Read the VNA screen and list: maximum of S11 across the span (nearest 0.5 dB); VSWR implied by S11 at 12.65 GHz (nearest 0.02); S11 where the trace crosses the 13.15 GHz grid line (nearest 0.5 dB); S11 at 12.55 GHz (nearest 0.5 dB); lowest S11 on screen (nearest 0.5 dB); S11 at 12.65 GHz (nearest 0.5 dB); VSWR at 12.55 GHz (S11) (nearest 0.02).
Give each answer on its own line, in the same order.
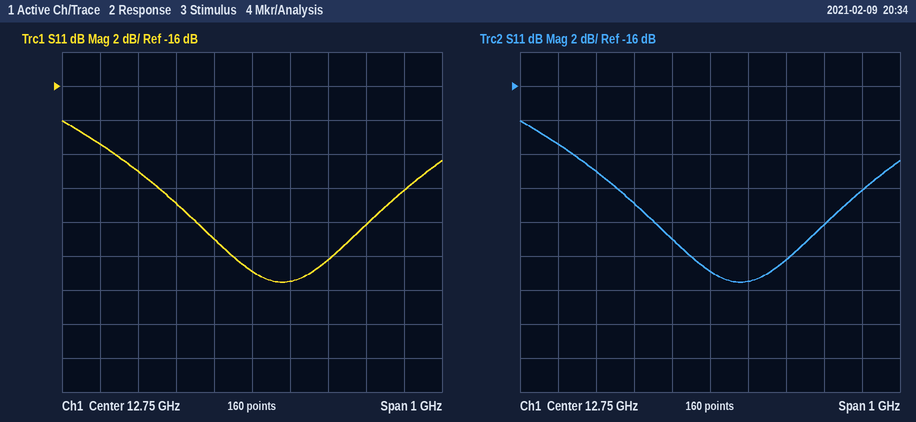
-18.0 dB
1.12
-22.0 dB
-23.0 dB
-27.5 dB
-25.0 dB
1.16
